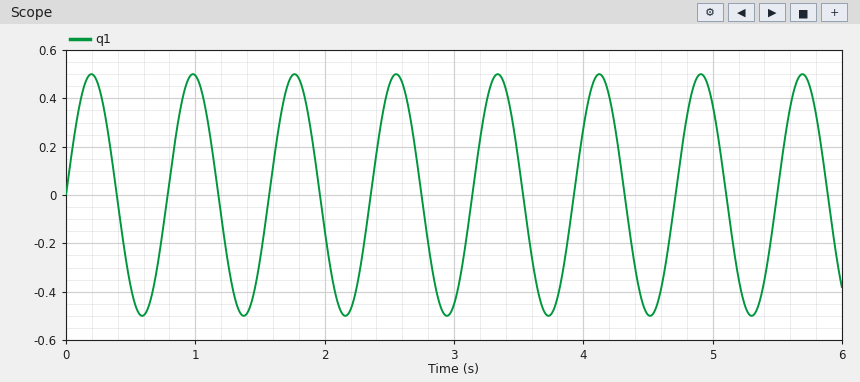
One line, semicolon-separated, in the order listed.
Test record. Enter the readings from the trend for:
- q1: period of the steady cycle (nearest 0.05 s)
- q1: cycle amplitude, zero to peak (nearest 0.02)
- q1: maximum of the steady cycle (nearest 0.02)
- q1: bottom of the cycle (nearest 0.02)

0.80 s; 0.50; 0.50; -0.50
